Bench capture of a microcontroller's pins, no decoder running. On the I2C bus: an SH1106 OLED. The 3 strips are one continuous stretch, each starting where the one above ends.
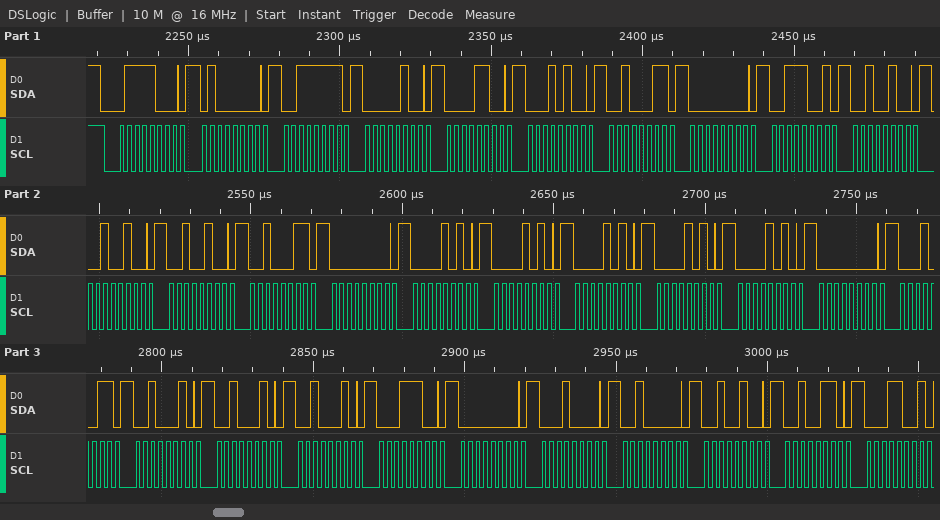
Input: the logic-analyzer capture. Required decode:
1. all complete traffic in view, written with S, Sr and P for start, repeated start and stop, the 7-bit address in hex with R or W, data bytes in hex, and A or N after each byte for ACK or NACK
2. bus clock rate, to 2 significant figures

S 3CW A 40 A 3F A 04 A 0C A 14 A 23 A 00 A 39 A 24 A 24 A 24 A 23 A 00 A 0A A 0A A 0A A 0A A 0A A 00 A 13 A 22 A 22 A 22 A 1C A 00 A 10 A 20 A 24 A 26 A 19 A
400 kHz
